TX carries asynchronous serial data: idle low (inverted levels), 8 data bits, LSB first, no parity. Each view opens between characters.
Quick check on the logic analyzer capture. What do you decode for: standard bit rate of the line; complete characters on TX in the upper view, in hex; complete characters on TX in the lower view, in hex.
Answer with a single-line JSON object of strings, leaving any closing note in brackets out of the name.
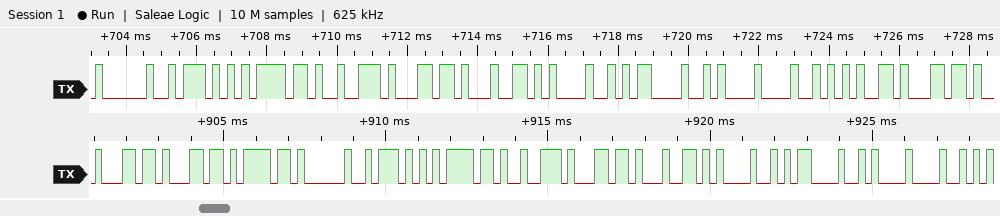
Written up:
{"standard bit rate of the line": "4800 baud", "complete characters on TX in the upper view, in hex": "BF, 51, 21, 1B, 27, 37, BD, E5, EB, 6F, 35, 27", "complete characters on TX in the lower view, in hex": "27, 27, 21, BF, 51, 21, 1B, 27, 37, BD, E5, EB, 6F"}
